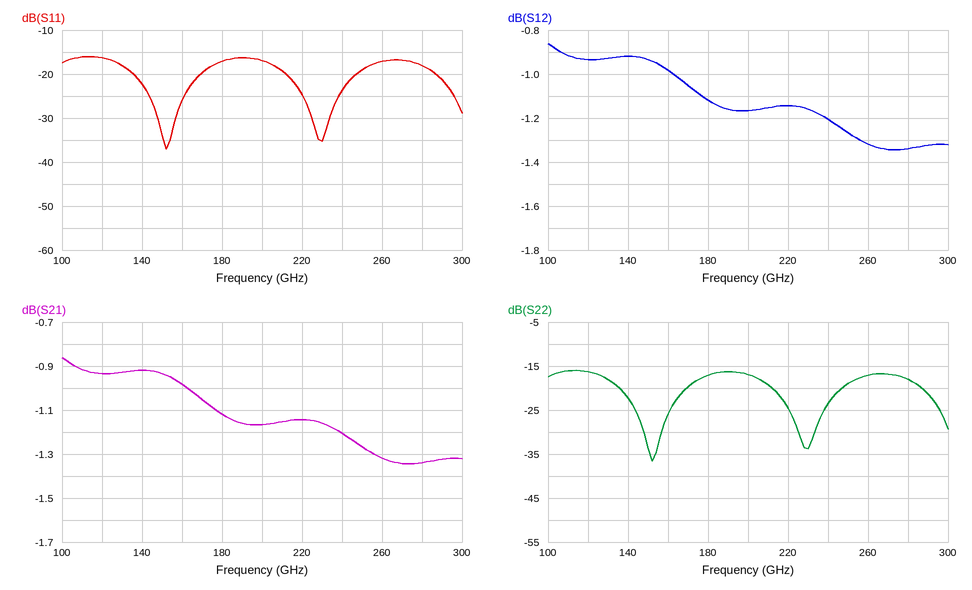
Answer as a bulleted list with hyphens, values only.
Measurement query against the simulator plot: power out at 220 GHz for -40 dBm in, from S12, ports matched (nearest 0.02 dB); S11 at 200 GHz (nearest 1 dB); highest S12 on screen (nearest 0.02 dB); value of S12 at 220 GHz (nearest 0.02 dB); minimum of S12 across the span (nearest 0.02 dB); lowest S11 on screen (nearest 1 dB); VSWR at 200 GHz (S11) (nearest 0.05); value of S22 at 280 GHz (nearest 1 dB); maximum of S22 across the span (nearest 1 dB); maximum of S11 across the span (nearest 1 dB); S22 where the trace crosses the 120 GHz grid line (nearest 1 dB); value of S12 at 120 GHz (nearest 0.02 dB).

- -41.14 dBm
- -17 dB
- -0.86 dB
- -1.14 dB
- -1.34 dB
- -37 dB
- 1.35
- -18 dB
- -16 dB
- -16 dB
- -16 dB
- -0.94 dB
